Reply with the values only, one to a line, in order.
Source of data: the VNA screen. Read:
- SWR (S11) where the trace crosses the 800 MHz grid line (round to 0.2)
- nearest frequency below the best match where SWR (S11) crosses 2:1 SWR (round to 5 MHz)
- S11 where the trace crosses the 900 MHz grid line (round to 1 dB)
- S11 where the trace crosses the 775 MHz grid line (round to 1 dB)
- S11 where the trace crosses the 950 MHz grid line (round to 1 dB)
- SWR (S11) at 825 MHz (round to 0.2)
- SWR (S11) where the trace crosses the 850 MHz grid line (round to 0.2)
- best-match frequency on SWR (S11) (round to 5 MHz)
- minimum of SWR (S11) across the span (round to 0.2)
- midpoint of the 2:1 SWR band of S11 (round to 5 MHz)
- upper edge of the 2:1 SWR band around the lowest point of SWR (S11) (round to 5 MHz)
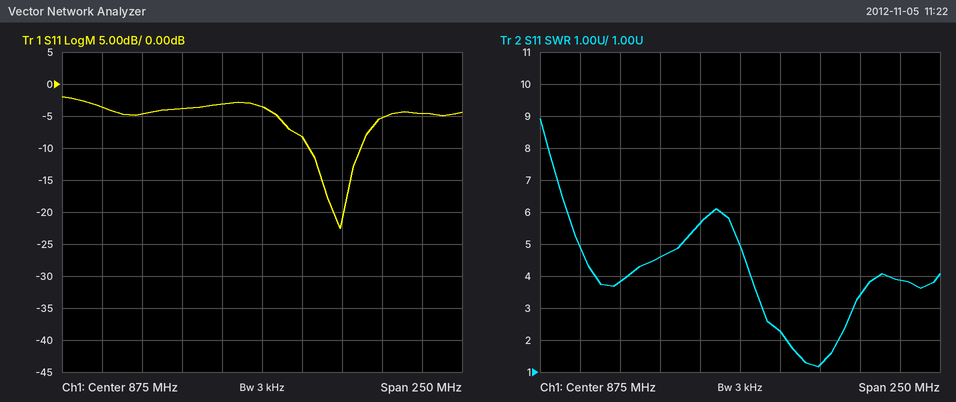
3.8
905 MHz
-8 dB
-4 dB
-5 dB
4.6
5.6
925 MHz
1.2
920 MHz
935 MHz
